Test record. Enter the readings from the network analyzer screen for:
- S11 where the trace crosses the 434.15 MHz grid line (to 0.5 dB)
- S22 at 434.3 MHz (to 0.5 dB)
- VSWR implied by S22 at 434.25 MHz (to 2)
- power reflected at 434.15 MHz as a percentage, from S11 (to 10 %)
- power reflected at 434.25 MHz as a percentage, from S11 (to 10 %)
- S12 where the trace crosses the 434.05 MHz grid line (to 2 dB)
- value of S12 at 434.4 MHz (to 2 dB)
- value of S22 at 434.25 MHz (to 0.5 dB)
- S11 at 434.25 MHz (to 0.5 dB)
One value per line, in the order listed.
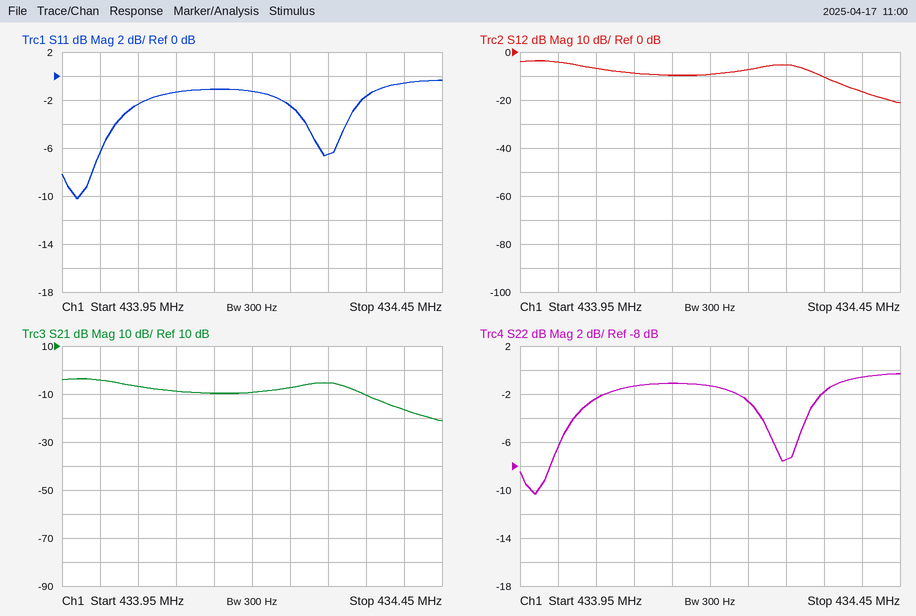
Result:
-1.0 dB
-7.5 dB
6
80 %
60 %
-6 dB
-16 dB
-2.5 dB
-2.5 dB
